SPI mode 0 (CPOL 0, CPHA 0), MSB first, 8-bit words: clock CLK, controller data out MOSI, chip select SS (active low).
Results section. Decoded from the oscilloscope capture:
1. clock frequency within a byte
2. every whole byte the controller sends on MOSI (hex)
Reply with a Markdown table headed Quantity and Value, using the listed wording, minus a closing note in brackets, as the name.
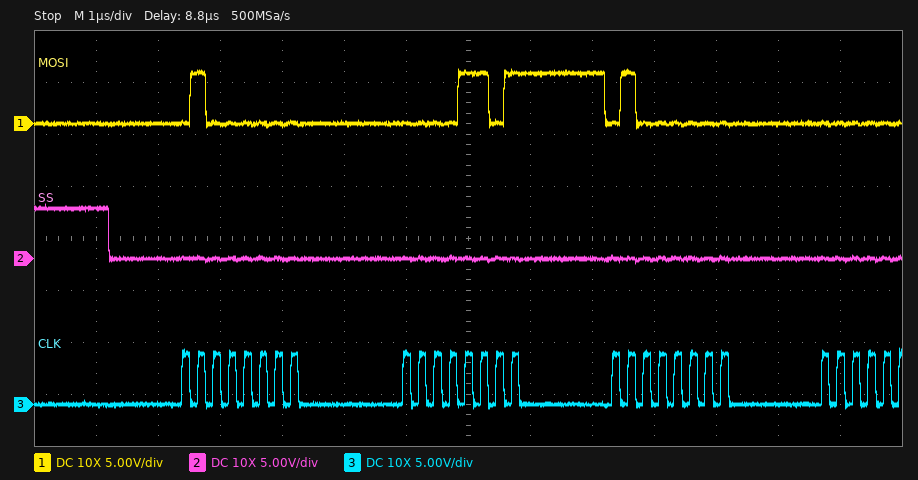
| Quantity | Value |
|---|---|
| clock frequency within a byte | 4 MHz |
| every whole byte the controller sends on MOSI | 0x40 0x0D 0x40 |
